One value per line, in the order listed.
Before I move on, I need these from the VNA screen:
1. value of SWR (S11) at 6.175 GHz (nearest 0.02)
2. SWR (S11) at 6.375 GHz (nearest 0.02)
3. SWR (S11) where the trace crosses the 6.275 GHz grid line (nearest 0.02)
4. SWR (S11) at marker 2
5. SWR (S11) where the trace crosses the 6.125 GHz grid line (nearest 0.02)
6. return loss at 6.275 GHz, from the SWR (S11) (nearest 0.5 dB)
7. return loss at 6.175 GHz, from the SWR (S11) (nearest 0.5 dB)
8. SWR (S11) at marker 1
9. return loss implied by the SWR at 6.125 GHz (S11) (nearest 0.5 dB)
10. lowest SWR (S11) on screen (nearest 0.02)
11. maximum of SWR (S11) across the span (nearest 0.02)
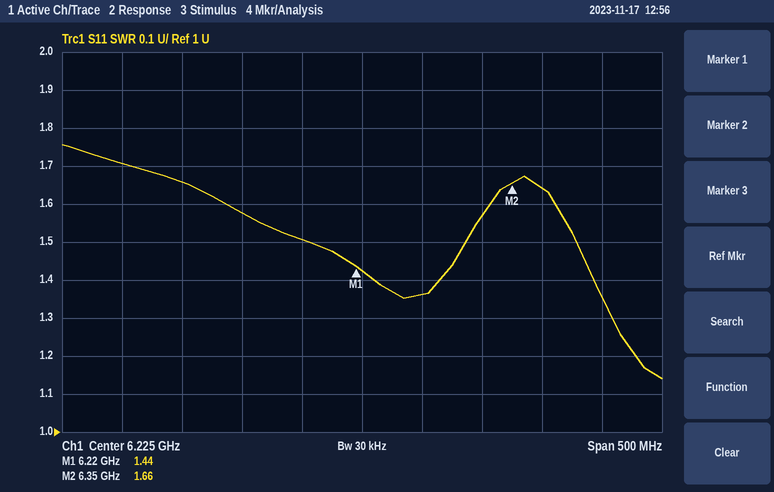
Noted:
1.50
1.64
1.36
1.66
1.58
16.5 dB
14.0 dB
1.44
13.0 dB
1.14
1.76
